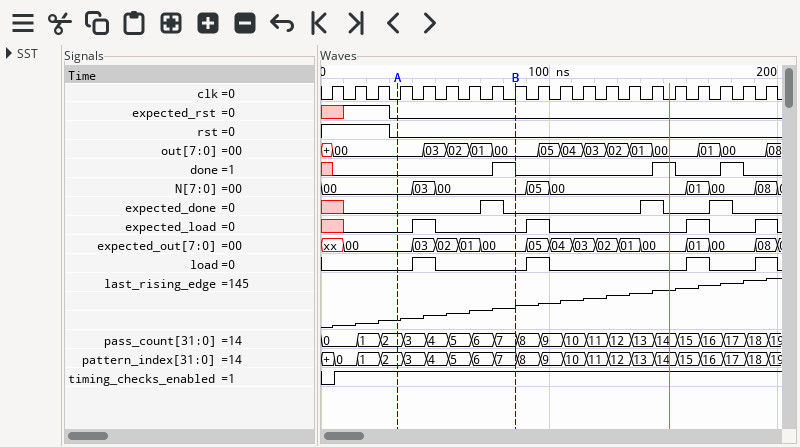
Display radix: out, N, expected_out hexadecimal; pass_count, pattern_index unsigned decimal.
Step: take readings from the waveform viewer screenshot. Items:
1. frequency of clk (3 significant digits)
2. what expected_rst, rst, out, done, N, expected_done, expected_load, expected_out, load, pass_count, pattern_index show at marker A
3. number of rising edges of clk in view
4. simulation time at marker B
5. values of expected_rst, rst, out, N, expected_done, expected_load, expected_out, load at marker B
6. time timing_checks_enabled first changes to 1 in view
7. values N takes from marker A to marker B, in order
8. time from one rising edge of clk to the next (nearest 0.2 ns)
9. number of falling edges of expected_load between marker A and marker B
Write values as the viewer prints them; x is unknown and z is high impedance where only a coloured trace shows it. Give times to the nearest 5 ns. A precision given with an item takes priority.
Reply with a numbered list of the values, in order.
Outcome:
1. 100 MHz
2. expected_rst=0, rst=0, out=00, done=0, N=00, expected_done=0, expected_load=0, expected_out=00, load=0, pass_count=2, pattern_index=2
3. 20
4. 85 ns
5. expected_rst=0, rst=0, out=00, N=00, expected_done=0, expected_load=0, expected_out=00, load=0
6. 5 ns
7. 00, 03, 00
8. 10 ns
9. 1
